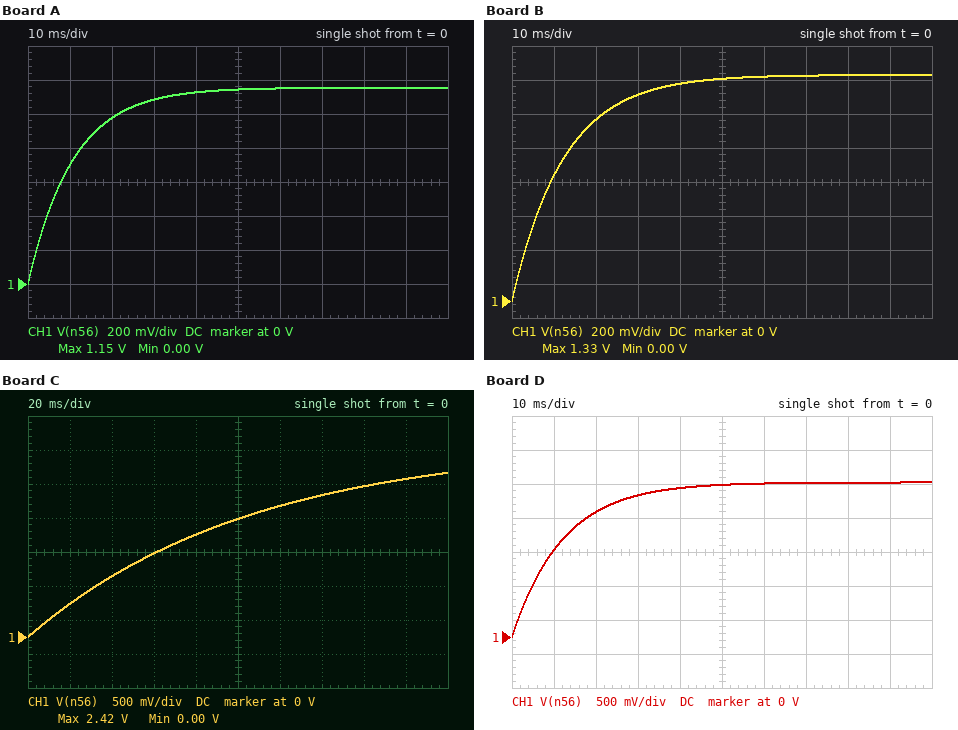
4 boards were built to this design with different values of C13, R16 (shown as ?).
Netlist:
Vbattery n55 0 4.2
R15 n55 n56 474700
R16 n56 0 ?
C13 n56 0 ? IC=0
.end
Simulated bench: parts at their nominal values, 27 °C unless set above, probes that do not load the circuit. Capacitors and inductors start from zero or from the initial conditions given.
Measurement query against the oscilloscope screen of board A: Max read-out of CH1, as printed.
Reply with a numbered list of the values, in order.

1. 1.15 V
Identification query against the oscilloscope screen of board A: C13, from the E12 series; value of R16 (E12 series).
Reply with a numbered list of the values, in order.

1. 82 nF
2. 180 kΩ
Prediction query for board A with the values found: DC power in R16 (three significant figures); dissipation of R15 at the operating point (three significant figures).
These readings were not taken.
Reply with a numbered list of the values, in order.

1. 7.41 µW
2. 19.5 µW
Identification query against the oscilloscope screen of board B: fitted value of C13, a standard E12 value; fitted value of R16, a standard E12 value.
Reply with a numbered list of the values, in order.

1. 82 nF
2. 220 kΩ
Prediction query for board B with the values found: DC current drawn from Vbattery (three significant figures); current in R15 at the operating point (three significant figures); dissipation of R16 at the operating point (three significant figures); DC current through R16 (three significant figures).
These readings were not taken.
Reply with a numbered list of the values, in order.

1. 6.05 µA
2. 6.05 µA
3. 8.04 µW
4. 6.05 µA
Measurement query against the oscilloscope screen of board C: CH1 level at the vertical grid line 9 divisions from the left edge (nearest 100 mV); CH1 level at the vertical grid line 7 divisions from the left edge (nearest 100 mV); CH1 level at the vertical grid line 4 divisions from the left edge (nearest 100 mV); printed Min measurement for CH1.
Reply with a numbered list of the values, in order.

1. 2.3 V
2. 2.1 V
3. 1.5 V
4. 0.00 V
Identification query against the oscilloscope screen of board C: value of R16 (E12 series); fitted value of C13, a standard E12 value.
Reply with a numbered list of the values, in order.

1. 1 MΩ
2. 330 nF
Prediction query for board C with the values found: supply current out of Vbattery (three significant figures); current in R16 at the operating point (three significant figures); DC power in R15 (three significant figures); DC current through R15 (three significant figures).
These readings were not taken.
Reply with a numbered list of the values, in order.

1. 2.85 µA
2. 2.85 µA
3. 3.85 µW
4. 2.85 µA
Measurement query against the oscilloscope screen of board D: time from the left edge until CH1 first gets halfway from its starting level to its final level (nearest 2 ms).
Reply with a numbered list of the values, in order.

1. 8 ms
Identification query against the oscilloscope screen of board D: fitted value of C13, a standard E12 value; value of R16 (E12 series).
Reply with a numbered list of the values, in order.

1. 47 nF
2. 560 kΩ
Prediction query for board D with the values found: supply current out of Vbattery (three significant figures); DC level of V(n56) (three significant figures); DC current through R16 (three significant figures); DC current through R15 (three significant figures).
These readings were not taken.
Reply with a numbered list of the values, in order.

1. 4.06 µA
2. 2.27 V
3. 4.06 µA
4. 4.06 µA
